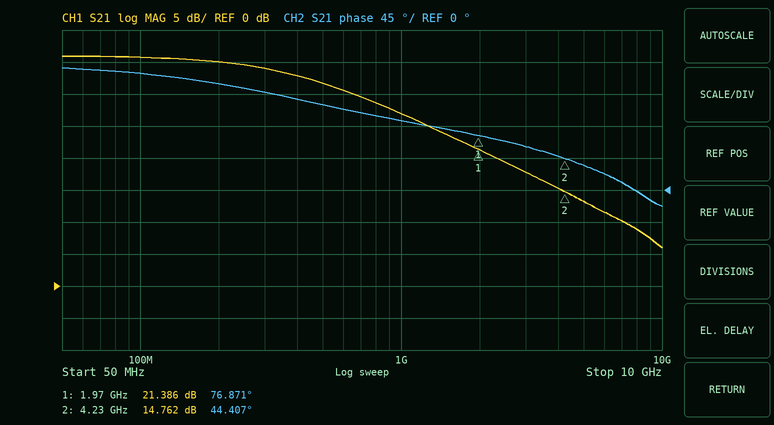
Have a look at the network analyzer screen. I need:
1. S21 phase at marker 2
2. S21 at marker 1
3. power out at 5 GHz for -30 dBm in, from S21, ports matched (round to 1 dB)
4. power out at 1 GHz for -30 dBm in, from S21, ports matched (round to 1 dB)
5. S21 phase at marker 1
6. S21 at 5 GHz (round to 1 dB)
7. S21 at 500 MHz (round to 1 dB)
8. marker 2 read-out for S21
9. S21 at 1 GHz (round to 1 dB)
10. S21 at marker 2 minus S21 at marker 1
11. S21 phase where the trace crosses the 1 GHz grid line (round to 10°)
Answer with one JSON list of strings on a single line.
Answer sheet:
["44.407°", "21.386 dB", "-17 dBm", "-3 dBm", "76.871°", "13 dB", "32 dB", "14.762 dB", "27 dB", "-6.624 dB", "100°"]
